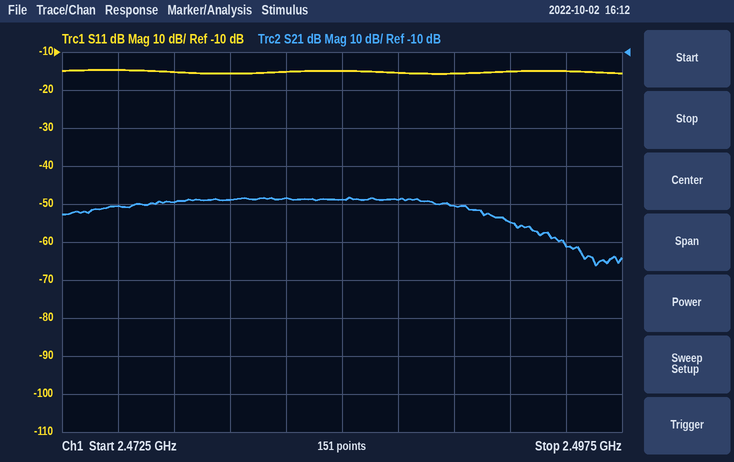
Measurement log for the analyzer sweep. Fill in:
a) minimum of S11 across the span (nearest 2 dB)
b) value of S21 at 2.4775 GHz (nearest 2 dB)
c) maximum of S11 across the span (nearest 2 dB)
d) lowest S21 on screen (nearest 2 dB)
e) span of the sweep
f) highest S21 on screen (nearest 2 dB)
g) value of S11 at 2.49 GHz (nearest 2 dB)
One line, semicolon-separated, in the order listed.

-16 dB; -50 dB; -14 dB; -66 dB; 25 MHz; -48 dB; -16 dB
